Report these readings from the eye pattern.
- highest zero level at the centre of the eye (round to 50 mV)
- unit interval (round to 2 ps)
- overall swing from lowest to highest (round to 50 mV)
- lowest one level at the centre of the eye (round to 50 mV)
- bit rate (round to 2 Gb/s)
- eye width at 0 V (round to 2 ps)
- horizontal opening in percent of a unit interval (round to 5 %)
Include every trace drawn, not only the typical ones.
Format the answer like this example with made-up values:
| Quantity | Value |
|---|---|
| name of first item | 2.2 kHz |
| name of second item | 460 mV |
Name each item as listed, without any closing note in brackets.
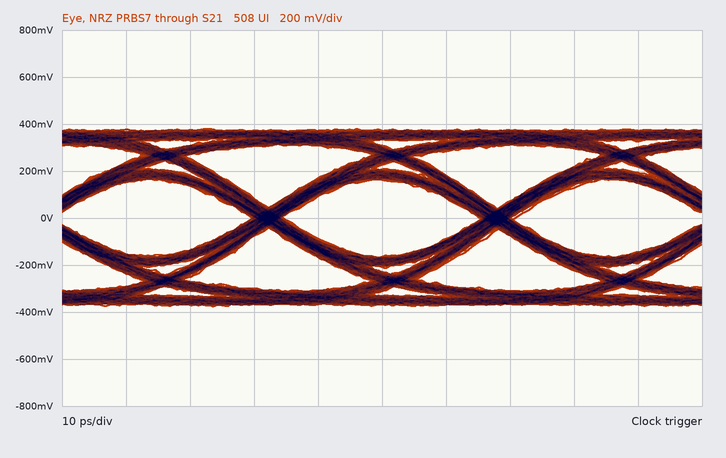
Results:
| Quantity | Value |
|---|---|
| highest zero level at the centre of the eye | -150 mV |
| unit interval | 36 ps |
| overall swing from lowest to highest | 750 mV |
| lowest one level at the centre of the eye | 150 mV |
| bit rate | 28 Gb/s |
| eye width at 0 V | 30 ps |
| horizontal opening in percent of a unit interval | 85 % |
